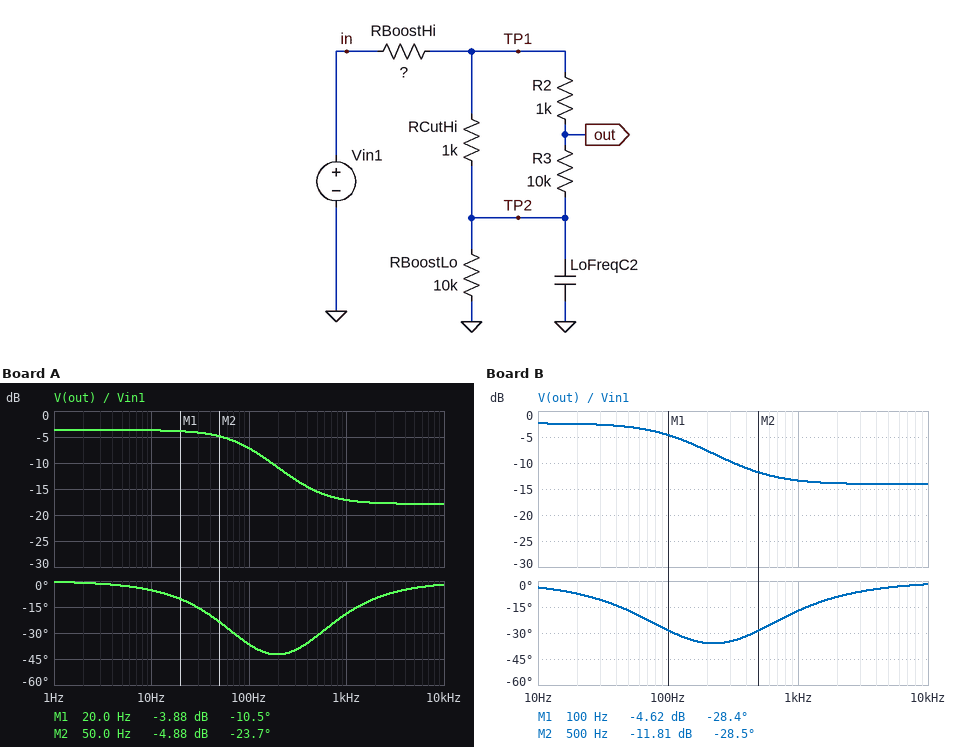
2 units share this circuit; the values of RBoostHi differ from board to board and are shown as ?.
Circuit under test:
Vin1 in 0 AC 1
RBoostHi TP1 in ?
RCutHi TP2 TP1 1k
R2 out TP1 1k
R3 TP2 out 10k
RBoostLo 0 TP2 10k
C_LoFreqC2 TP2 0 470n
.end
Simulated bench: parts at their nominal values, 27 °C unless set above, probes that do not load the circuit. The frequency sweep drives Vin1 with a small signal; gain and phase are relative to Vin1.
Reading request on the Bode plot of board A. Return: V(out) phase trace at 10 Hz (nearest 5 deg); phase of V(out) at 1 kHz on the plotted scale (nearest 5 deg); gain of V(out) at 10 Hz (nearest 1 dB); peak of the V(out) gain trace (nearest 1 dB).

-5 deg
-20 deg
-4 dB
-4 dB
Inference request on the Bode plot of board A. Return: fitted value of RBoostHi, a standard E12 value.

5.6 kΩ
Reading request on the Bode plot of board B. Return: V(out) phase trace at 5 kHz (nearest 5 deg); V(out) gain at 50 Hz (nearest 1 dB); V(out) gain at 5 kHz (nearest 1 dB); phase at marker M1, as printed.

-5 deg
-3 dB
-14 dB
-28.4 deg
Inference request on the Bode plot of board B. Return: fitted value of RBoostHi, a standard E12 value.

3.3 kΩ
